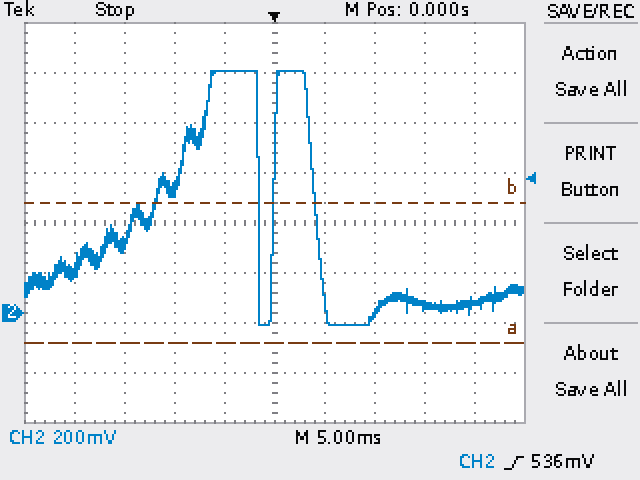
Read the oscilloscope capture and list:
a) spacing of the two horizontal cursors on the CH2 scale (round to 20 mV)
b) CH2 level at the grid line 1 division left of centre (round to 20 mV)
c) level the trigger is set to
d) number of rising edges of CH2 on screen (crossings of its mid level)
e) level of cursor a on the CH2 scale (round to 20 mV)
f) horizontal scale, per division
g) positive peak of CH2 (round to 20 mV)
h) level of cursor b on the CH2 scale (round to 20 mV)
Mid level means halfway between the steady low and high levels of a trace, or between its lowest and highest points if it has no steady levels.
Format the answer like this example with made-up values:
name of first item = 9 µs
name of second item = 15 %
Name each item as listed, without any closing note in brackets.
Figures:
spacing of the two horizontal cursors on the CH2 scale = 560 mV
CH2 level at the grid line 1 division left of centre = 960 mV
level the trigger is set to = 536 mV
number of rising edges of CH2 on screen = 2
level of cursor a on the CH2 scale = -120 mV
horizontal scale, per division = 5 ms
positive peak of CH2 = 960 mV
level of cursor b on the CH2 scale = 440 mV
